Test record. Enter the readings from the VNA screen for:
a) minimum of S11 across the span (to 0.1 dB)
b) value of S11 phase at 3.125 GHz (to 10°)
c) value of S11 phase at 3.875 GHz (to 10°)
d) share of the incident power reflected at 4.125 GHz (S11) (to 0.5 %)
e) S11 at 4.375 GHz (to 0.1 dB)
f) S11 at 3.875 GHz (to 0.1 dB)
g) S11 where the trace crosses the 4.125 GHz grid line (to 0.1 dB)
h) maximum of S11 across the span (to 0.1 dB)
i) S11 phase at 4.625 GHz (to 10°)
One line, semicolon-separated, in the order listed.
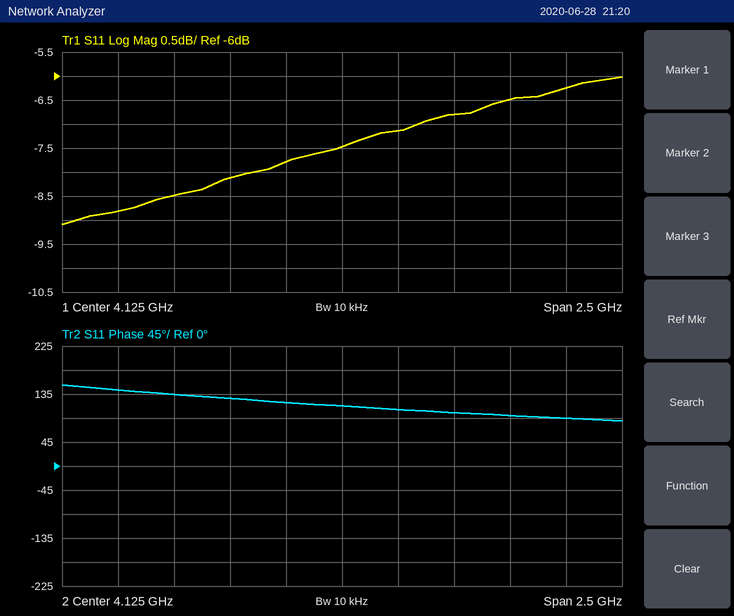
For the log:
-9.1 dB; 140°; 120°; 18.0 %; -7.1 dB; -7.8 dB; -7.5 dB; -6.0 dB; 100°
